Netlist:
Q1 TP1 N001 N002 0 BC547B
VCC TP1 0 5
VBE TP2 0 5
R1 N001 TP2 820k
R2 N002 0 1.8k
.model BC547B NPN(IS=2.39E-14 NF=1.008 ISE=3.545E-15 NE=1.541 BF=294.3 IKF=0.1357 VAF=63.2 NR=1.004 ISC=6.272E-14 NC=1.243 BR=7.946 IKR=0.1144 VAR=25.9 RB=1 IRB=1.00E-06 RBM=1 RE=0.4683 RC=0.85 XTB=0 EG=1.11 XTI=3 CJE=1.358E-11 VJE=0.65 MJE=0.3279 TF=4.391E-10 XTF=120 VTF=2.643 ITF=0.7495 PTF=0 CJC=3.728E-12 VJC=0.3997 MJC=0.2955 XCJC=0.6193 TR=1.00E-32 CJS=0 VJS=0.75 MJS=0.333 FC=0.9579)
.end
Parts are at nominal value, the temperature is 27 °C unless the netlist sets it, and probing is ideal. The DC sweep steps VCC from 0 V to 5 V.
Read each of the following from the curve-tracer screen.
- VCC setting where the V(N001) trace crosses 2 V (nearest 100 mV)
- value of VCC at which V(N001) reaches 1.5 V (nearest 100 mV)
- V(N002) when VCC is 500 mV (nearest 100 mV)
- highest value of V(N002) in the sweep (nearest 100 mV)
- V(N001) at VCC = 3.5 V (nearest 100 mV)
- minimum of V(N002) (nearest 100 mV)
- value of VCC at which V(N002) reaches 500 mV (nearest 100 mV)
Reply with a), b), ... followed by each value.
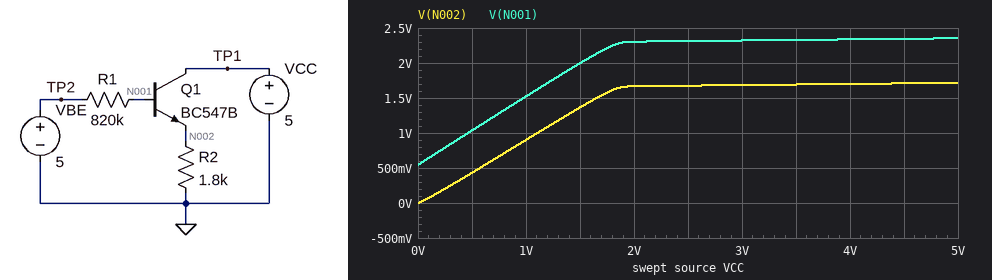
a) 1.5 V
b) 1.0 V
c) 400 mV
d) 1.7 V
e) 2.3 V
f) 0 V
g) 600 mV
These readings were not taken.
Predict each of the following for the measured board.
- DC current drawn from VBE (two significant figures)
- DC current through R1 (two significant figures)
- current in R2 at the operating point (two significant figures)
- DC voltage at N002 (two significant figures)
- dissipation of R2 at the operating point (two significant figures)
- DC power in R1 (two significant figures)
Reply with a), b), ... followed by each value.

a) 3.2 µA
b) 3.2 µA
c) 950 µA
d) 1.7 V
e) 1.6 mW
f) 8.5 µW
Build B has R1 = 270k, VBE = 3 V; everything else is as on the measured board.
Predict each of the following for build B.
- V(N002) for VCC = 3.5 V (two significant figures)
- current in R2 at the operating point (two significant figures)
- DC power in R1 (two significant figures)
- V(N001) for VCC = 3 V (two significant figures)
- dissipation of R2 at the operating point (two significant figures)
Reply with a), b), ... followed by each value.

a) 1.6 V
b) 870 µA
c) 2.3 µW
d) 2.2 V
e) 1.4 mW
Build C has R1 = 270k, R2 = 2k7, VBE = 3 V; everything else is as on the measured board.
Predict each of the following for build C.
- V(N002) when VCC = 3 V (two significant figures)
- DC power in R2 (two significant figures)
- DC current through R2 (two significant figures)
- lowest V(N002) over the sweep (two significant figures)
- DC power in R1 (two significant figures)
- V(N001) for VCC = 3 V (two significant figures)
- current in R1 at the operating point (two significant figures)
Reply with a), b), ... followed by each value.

a) 1.8 V
b) 1.2 mW
c) 660 µA
d) -1.8 mV
e) 1.3 µW
f) 2.4 V
g) 2.2 µA
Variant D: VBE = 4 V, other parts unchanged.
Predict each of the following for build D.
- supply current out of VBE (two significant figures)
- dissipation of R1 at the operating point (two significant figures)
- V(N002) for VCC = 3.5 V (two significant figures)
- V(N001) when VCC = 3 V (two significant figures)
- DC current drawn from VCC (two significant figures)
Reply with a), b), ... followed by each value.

a) 2.5 µA
b) 5.1 µW
c) 1.3 V
d) 1.9 V
e) 740 µA
